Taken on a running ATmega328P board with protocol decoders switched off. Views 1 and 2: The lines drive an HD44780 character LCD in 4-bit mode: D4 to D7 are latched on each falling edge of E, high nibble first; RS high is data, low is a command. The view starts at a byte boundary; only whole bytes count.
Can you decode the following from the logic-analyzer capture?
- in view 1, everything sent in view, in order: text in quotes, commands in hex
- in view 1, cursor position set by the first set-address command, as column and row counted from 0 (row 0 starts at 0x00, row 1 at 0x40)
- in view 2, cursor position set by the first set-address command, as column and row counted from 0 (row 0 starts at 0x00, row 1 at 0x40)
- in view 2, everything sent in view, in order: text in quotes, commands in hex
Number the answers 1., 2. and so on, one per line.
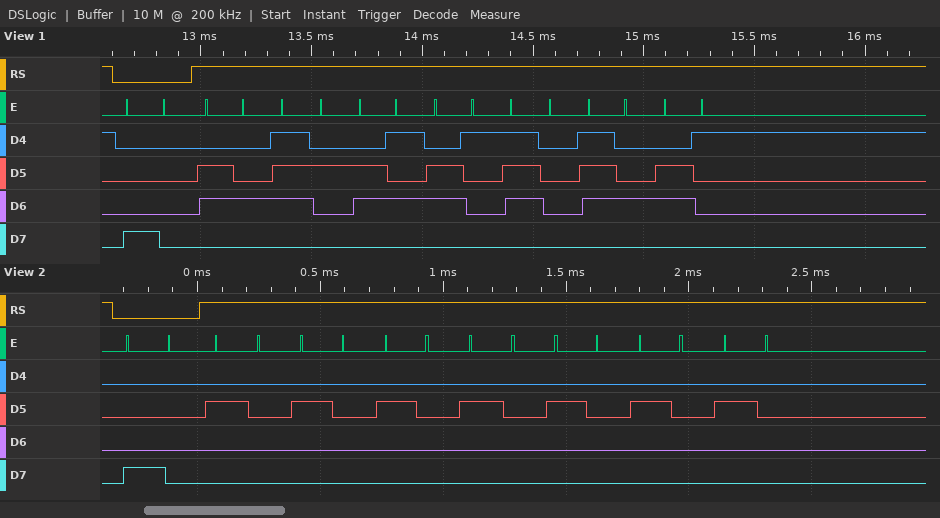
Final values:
1. 0x80 "dreapta"
2. column 0, row 0
3. column 0, row 0
4. 0x80 "       "
